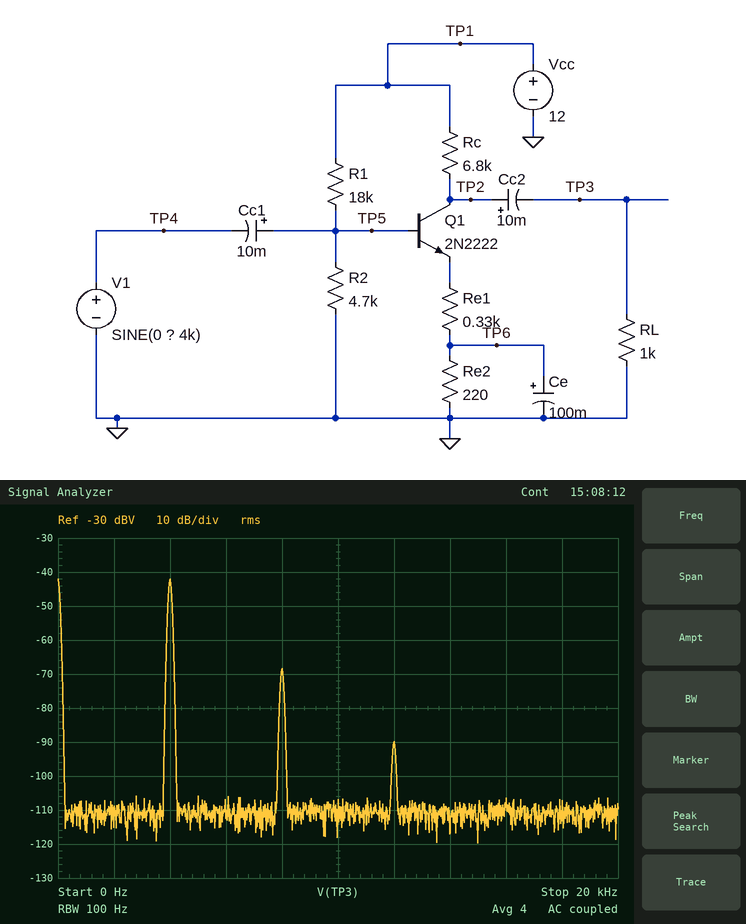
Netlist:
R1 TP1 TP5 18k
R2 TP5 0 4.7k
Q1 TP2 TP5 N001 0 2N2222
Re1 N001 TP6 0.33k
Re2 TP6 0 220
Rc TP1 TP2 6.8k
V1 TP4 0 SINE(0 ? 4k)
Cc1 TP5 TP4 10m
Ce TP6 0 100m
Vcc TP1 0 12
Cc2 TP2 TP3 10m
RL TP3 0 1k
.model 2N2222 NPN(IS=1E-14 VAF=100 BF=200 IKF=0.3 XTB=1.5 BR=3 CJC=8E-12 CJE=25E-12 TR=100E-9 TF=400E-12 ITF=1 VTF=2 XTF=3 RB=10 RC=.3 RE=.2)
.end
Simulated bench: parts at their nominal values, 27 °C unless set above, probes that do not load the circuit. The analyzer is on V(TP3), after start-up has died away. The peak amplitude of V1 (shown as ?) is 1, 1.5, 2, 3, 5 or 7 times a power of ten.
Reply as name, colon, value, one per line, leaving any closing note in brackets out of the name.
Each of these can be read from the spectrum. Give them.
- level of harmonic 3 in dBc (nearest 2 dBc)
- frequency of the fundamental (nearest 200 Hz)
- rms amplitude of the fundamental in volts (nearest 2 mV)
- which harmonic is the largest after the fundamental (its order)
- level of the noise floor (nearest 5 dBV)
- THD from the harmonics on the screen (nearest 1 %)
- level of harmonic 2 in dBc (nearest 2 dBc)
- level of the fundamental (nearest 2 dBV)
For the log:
level of harmonic 3 in dBc: -48 dBc
frequency of the fundamental: 4.0 kHz
rms amplitude of the fundamental in volts: 8 mV
which harmonic is the largest after the fundamental: 2
level of the noise floor: -110 dBV
THD from the harmonics on the screen: 5 %
level of harmonic 2 in dBc: -26 dBc
level of the fundamental: -42 dBV
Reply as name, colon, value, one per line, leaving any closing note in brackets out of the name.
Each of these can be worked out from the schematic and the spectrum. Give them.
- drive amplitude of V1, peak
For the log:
drive amplitude of V1, peak: 20 mV
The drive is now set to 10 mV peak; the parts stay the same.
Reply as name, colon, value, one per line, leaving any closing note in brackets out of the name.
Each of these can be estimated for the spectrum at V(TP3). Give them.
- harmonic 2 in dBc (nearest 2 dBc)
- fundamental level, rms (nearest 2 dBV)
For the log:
harmonic 2 in dBc: -32 dBc
fundamental level, rms: -48 dBV
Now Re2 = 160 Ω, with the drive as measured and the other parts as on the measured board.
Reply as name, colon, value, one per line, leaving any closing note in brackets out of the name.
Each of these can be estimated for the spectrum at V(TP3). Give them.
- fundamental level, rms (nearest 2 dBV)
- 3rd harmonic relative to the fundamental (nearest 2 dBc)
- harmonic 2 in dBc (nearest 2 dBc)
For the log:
fundamental level, rms: -42 dBV
3rd harmonic relative to the fundamental: -50 dBc
harmonic 2 in dBc: -28 dBc
